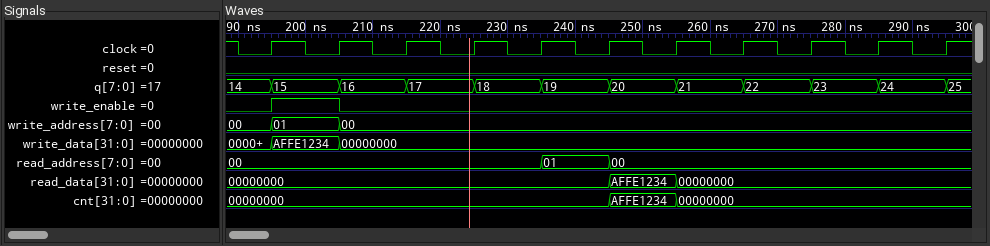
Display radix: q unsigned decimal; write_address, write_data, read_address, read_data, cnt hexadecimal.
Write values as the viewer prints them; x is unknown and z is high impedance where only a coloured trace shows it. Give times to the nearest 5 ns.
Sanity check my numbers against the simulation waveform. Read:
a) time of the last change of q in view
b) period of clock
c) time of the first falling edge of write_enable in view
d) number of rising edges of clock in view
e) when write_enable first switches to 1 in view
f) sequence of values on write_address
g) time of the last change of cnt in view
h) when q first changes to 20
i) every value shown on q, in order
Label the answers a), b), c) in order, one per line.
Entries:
a) 295 ns
b) 10 ns
c) 205 ns
d) 11
e) 195 ns
f) 00, 01, 00
g) 255 ns
h) 245 ns
i) 14, 15, 16, 17, 18, 19, 20, 21, 22, 23, 24, 25
